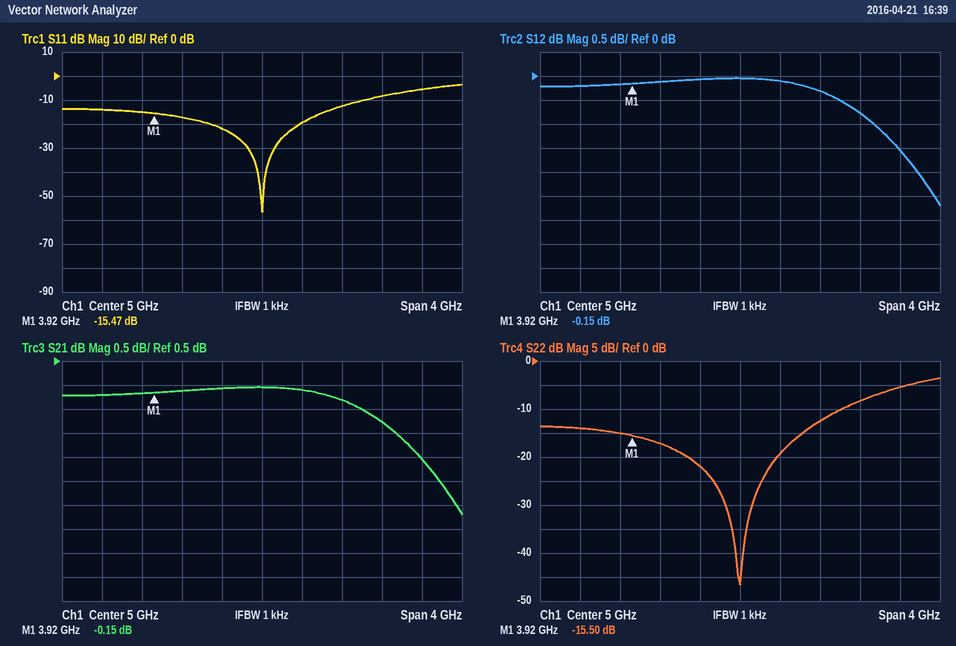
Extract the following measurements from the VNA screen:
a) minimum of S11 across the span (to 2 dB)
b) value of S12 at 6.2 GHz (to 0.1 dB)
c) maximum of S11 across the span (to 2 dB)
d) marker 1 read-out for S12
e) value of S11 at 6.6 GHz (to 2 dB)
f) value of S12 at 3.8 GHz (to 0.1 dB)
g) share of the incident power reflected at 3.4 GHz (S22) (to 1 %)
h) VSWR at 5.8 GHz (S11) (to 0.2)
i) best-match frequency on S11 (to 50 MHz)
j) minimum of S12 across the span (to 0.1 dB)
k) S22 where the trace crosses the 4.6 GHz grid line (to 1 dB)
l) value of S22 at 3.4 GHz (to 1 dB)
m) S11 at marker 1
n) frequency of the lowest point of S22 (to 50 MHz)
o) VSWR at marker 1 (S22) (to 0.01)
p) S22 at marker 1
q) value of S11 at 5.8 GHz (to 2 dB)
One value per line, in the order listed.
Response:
-56 dB
-0.8 dB
-4 dB
-0.15 dB
-6 dB
-0.2 dB
4 %
1.6
5.00 GHz
-2.7 dB
-22 dB
-14 dB
-15.47 dB
5.00 GHz
1.40
-15.50 dB
-12 dB
